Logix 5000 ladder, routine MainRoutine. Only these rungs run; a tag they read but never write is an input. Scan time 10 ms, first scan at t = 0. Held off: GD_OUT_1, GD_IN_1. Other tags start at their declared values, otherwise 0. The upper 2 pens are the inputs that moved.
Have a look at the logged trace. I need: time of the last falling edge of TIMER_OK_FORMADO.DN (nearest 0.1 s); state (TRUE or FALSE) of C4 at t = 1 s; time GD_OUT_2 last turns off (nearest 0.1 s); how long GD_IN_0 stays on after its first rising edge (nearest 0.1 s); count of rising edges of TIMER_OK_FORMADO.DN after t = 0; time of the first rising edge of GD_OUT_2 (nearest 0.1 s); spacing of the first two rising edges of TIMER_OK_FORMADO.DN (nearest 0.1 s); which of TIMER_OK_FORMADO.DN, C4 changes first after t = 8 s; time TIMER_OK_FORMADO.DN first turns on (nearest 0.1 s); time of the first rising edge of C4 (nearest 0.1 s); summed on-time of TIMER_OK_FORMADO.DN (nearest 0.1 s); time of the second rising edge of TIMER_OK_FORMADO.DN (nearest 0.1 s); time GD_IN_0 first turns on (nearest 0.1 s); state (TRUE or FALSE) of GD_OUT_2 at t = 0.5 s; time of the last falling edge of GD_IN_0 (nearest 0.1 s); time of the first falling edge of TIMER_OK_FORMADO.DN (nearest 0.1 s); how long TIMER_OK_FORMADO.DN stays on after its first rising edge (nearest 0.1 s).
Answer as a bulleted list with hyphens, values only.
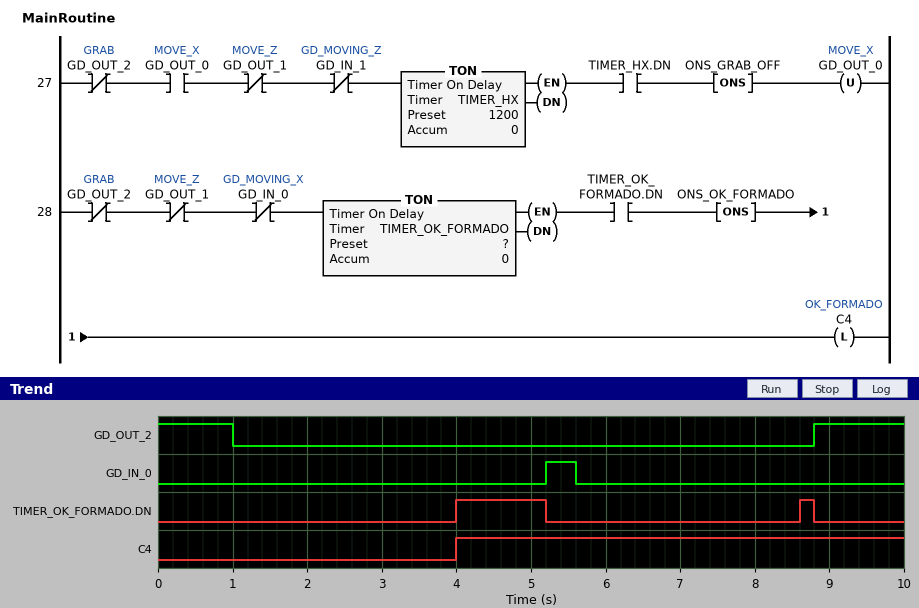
- 8.8 s
- FALSE
- 1.0 s
- 0.4 s
- 2
- 8.8 s
- 4.6 s
- TIMER_OK_FORMADO.DN
- 4.0 s
- 4.0 s
- 1.4 s
- 8.6 s
- 5.2 s
- TRUE
- 5.6 s
- 5.2 s
- 1.2 s
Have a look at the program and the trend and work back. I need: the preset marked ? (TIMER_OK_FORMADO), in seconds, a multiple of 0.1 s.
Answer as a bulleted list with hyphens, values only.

- 3.0 s
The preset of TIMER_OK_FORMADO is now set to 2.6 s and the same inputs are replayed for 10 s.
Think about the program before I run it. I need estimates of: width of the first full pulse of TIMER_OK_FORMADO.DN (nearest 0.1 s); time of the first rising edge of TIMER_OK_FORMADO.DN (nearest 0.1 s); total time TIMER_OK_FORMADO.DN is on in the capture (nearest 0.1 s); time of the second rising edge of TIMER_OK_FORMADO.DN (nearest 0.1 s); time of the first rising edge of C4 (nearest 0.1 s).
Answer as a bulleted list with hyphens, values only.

- 1.6 s
- 3.6 s
- 2.2 s
- 8.2 s
- 3.6 s
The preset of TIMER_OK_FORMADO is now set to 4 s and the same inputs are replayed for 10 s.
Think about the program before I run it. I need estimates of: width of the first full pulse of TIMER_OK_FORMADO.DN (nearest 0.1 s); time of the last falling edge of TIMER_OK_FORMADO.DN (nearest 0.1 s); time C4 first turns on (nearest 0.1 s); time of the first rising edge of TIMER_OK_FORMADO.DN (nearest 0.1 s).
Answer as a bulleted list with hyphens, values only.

- 0.2 s
- 5.2 s
- 5.0 s
- 5.0 s
